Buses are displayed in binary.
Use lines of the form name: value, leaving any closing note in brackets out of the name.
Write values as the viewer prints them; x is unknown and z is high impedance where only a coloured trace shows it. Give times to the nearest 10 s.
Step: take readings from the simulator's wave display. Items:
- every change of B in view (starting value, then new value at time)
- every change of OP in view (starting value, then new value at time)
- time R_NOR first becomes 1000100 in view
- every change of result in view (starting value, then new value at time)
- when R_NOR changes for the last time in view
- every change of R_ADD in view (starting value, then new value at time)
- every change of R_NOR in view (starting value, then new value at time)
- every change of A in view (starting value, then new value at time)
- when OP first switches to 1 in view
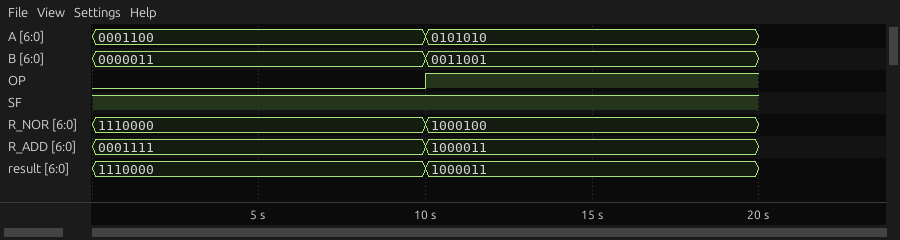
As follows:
every change of B in view: 0000011, 0011001 at 10 s
every change of OP in view: 0, 1 at 10 s
time R_NOR first becomes 1000100 in view: 10 s
every change of result in view: 1110000, 1000011 at 10 s
when R_NOR changes for the last time in view: 10 s
every change of R_ADD in view: 0001111, 1000011 at 10 s
every change of R_NOR in view: 1110000, 1000100 at 10 s
every change of A in view: 0001100, 0101010 at 10 s
when OP first switches to 1 in view: 10 s
